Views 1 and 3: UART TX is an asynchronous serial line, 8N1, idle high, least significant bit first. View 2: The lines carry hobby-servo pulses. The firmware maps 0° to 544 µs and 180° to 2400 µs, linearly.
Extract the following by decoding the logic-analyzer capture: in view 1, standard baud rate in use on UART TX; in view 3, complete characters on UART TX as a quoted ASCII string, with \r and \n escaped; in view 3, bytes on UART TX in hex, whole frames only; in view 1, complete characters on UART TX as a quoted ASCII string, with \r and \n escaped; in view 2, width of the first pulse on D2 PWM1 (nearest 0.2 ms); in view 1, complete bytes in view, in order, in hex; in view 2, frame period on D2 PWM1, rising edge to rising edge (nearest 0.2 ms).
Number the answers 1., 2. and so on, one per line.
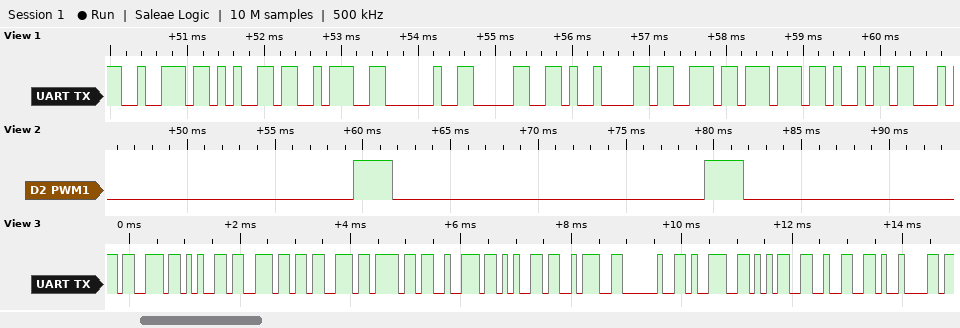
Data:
1. 9600 baud
2. "sensore: 952\t"
3. 73 65 6E 73 6F 72 65 3A 20 39 35 32 09
4. "re: 0\tswi"
5. 2.2 ms
6. 72 65 3A 20 30 09 73 77 69
7. 20.0 ms
